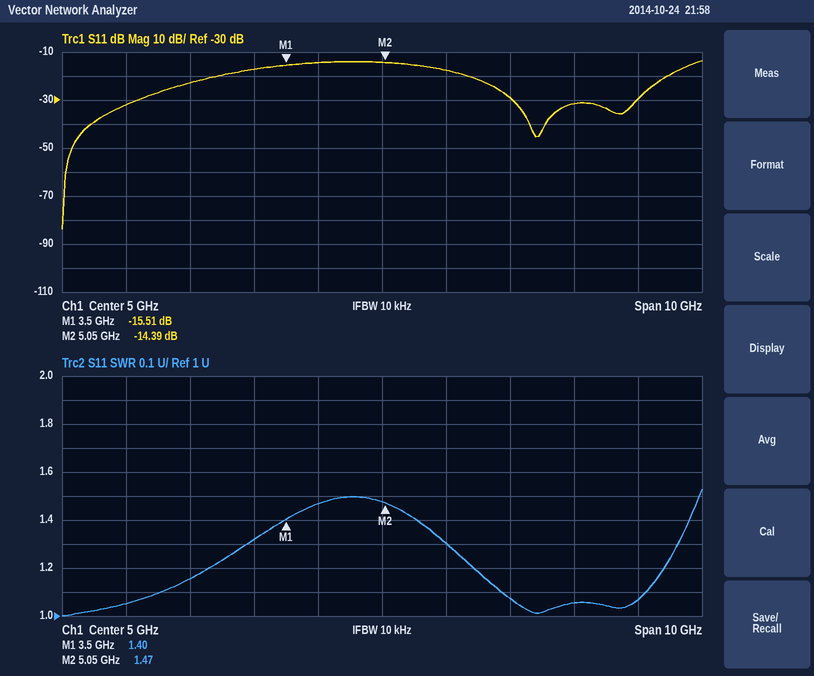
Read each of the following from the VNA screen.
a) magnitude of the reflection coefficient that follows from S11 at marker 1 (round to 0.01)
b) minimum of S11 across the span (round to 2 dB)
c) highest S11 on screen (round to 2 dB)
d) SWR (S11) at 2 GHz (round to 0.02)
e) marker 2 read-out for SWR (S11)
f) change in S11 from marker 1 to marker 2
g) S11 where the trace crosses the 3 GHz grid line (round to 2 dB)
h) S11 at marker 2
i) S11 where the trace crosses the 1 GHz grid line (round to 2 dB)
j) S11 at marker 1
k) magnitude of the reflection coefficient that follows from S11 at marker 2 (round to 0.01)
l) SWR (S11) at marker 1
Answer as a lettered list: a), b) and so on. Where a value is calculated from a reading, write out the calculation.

a) 10^(-15.51/20) ≈ 0.17
b) -84 dB
c) -14 dB
d) 1.16
e) 1.47
f) -14.39 − (-15.51) = 1.12 dB
g) -18 dB
h) -14.39 dB
i) -32 dB
j) -15.51 dB
k) 10^(-14.39/20) ≈ 0.19
l) 1.40
